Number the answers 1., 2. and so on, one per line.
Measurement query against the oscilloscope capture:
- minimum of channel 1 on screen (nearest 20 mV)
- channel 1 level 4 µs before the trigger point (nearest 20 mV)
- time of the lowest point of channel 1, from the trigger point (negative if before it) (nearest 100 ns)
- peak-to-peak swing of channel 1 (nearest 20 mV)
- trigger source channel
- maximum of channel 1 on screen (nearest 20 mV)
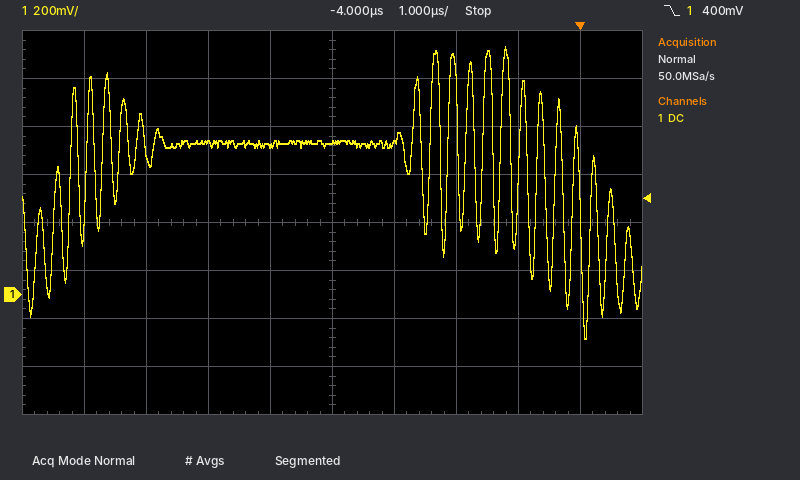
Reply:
1. -180 mV
2. 640 mV
3. +100 ns
4. 1.22 V
5. channel 1
6. 1.04 V
